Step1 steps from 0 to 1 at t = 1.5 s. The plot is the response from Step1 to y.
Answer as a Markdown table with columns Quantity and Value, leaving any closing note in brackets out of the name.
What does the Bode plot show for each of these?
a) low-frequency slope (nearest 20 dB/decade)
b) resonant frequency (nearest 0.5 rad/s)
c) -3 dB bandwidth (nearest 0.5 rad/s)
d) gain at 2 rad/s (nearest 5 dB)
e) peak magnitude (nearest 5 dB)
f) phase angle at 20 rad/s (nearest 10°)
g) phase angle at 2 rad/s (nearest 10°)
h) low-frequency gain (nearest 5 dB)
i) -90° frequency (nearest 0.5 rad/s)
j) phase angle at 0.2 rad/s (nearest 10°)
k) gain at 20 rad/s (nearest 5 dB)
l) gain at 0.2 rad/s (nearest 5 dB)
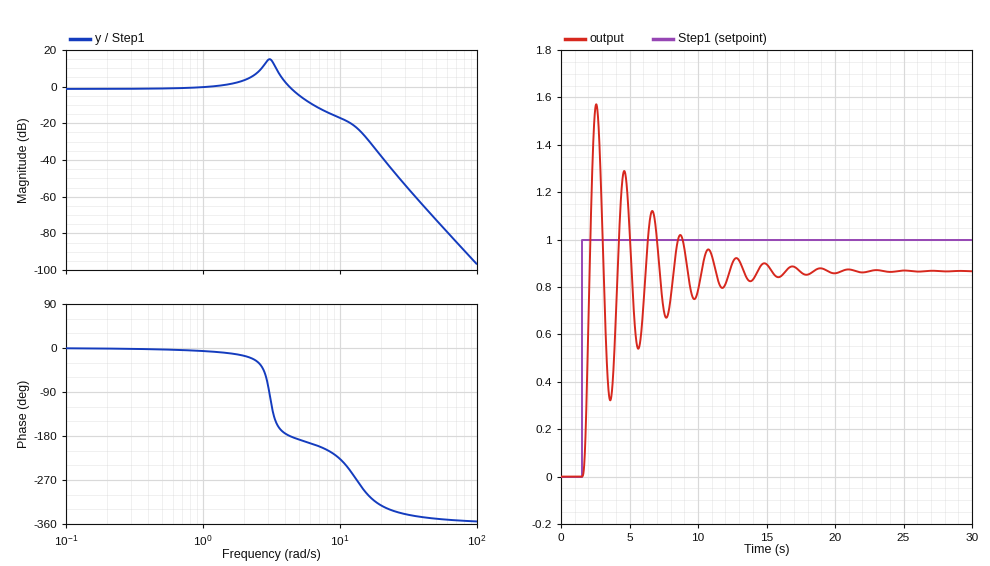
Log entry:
| Quantity | Value |
|---|---|
| low-frequency slope | 0 dB/decade |
| resonant frequency | 3.0 rad/s |
| -3 dB bandwidth | 5.0 rad/s |
| gain at 2 rad/s | 5 dB |
| peak magnitude | 15 dB |
| phase angle at 20 rad/s | -320° |
| phase angle at 2 rad/s | -20° |
| low-frequency gain | 0 dB |
| -90° frequency | 3.0 rad/s |
| phase angle at 0.2 rad/s | 0° |
| gain at 20 rad/s | -40 dB |
| gain at 0.2 rad/s | 0 dB |
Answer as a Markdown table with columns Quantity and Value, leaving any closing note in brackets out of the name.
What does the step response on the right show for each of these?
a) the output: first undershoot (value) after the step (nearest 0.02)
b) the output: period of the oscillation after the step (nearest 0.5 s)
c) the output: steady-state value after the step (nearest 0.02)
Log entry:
| Quantity | Value |
|---|---|
| the output: first undershoot (value) after the step | 0.32 |
| the output: period of the oscillation after the step | 2.0 s |
| the output: steady-state value after the step | 0.86 |
